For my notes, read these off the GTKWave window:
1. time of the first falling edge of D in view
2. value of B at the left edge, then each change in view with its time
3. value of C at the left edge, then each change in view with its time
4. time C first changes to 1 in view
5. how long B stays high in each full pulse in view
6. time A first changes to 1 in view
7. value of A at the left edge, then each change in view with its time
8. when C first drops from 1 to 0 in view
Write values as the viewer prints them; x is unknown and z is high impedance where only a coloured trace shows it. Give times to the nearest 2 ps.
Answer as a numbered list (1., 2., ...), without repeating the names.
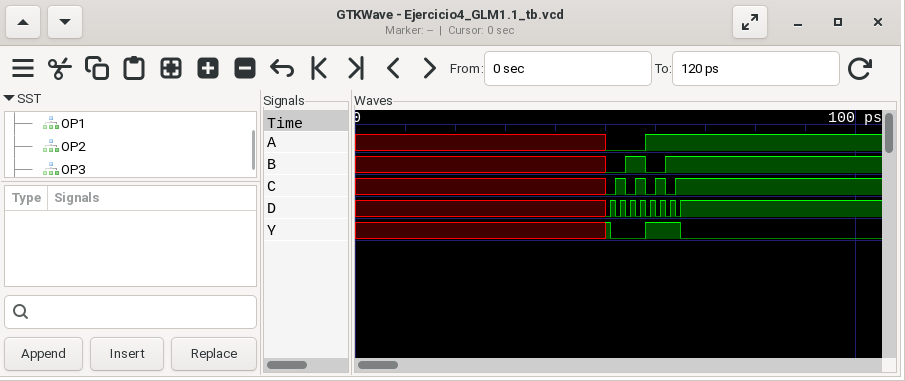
1. 52 ps
2. x, 0 at 50 ps, 1 at 54 ps, 0 at 58 ps, 1 at 62 ps
3. x, 0 at 50 ps, 1 at 52 ps, 0 at 54 ps, 1 at 56 ps, 0 at 58 ps, 1 at 60 ps, 0 at 62 ps, 1 at 64 ps
4. 52 ps
5. 4 ps
6. 58 ps
7. x, 0 at 50 ps, 1 at 58 ps
8. 54 ps
